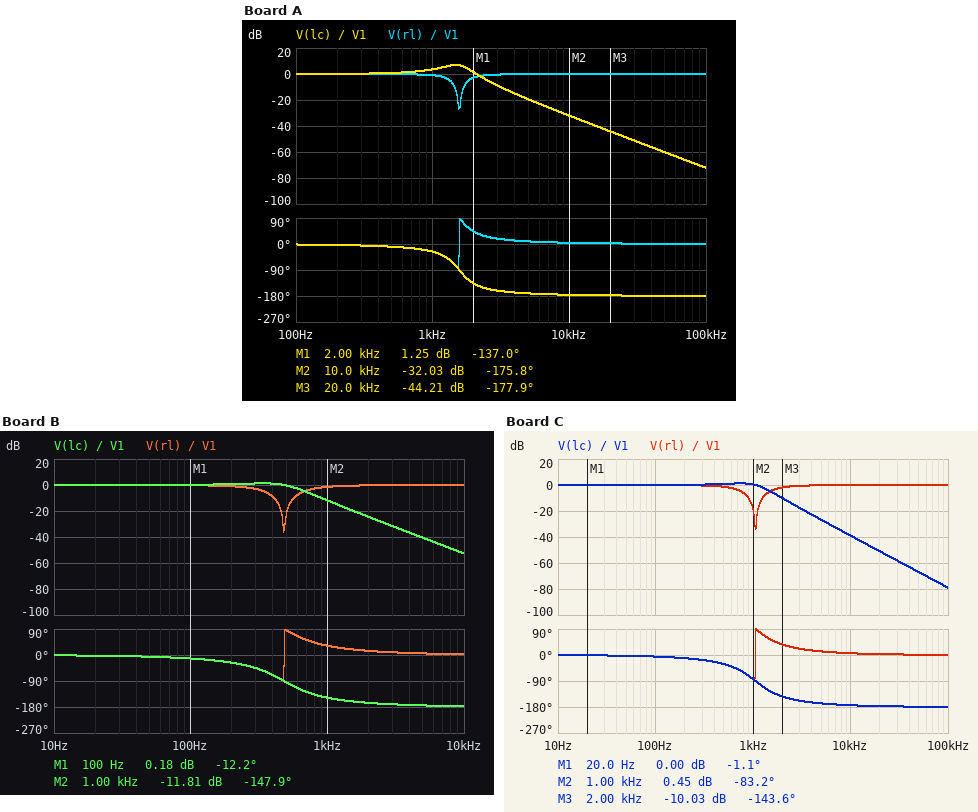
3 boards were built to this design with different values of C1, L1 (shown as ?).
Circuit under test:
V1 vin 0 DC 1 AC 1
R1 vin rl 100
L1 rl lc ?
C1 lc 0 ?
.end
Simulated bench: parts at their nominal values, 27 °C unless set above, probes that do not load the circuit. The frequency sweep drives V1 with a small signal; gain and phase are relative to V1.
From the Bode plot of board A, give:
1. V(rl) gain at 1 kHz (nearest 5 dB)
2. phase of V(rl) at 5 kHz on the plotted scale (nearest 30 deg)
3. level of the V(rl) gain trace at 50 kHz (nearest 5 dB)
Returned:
0 dB
0 deg
0 dB
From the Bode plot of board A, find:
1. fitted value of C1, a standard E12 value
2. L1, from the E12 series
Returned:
470 nF
22 mH
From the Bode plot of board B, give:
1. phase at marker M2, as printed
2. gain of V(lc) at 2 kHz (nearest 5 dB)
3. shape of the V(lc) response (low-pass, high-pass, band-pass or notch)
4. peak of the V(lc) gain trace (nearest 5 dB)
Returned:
-147.9 deg
-25 dB
low-pass
0 dB
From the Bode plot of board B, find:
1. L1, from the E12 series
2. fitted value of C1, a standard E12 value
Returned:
33 mH
3.3 µF
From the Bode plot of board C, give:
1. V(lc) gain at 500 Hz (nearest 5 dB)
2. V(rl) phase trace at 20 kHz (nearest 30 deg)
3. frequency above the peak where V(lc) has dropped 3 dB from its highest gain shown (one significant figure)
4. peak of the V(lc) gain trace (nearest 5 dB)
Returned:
0 dB
0 deg
1 kHz
0 dB
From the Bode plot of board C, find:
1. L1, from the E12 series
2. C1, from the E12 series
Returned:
15 mH
1.5 µF
